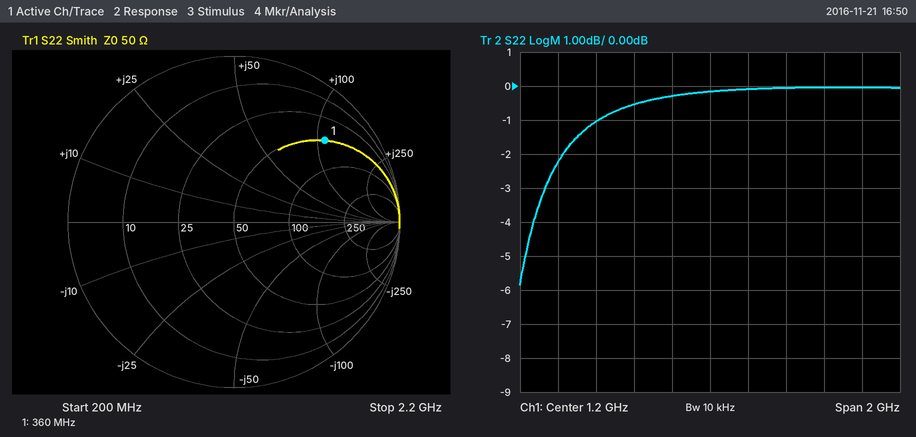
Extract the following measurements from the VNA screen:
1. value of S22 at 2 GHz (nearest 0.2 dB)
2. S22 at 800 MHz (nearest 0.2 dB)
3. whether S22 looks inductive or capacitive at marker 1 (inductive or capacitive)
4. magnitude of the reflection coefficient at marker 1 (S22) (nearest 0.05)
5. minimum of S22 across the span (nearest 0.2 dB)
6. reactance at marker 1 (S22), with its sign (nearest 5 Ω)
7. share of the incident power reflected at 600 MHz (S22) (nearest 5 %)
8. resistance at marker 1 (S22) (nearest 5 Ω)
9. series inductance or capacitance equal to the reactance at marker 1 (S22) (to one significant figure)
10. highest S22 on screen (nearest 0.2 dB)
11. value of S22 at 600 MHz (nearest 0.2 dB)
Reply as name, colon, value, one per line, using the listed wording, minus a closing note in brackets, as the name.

value of S22 at 2 GHz: 0.0 dB
S22 at 800 MHz: -0.6 dB
whether S22 looks inductive or capacitive at marker 1: inductive
magnitude of the reflection coefficient at marker 1 (S22): 0.75
minimum of S22 across the span: -5.8 dB
reactance at marker 1 (S22), with its sign: +110 Ω
share of the incident power reflected at 600 MHz (S22): 80 %
resistance at marker 1 (S22): 50 Ω
series inductance or capacitance equal to the reactance at marker 1 (S22): 50 nH
highest S22 on screen: 0.0 dB
value of S22 at 600 MHz: -1.0 dB
